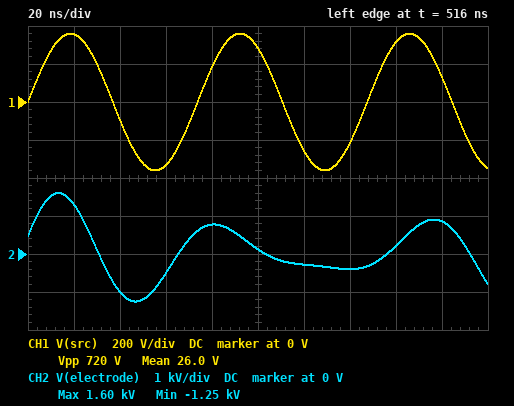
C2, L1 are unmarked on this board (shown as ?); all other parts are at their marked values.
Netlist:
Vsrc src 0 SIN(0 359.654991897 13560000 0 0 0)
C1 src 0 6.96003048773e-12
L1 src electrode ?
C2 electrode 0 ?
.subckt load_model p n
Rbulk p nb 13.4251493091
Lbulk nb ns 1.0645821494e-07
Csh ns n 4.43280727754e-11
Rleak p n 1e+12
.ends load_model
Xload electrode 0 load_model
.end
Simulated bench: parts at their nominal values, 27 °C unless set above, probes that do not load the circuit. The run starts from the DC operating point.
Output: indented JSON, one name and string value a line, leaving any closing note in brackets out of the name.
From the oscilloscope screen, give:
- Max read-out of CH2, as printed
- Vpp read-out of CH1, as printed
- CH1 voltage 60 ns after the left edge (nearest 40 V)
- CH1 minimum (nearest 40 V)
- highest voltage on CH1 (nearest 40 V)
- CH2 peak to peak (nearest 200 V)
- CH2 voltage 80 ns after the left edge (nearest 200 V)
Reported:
{
  "Max read-out of CH2, as printed": "1.60 kV",
  "Vpp read-out of CH1, as printed": "720 V",
  "CH1 voltage 60 ns after the left edge": "-320 V",
  "CH1 minimum": "-360 V",
  "highest voltage on CH1": "360 V",
  "CH2 peak to peak": "2.8 kV",
  "CH2 voltage 80 ns after the left edge": "800 V"
}
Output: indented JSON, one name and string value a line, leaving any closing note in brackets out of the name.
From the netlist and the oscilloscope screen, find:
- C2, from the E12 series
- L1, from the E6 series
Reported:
{
  "C2, from the E12 series": "560 pF",
  "L1, from the E6 series": "150 nH"
}
